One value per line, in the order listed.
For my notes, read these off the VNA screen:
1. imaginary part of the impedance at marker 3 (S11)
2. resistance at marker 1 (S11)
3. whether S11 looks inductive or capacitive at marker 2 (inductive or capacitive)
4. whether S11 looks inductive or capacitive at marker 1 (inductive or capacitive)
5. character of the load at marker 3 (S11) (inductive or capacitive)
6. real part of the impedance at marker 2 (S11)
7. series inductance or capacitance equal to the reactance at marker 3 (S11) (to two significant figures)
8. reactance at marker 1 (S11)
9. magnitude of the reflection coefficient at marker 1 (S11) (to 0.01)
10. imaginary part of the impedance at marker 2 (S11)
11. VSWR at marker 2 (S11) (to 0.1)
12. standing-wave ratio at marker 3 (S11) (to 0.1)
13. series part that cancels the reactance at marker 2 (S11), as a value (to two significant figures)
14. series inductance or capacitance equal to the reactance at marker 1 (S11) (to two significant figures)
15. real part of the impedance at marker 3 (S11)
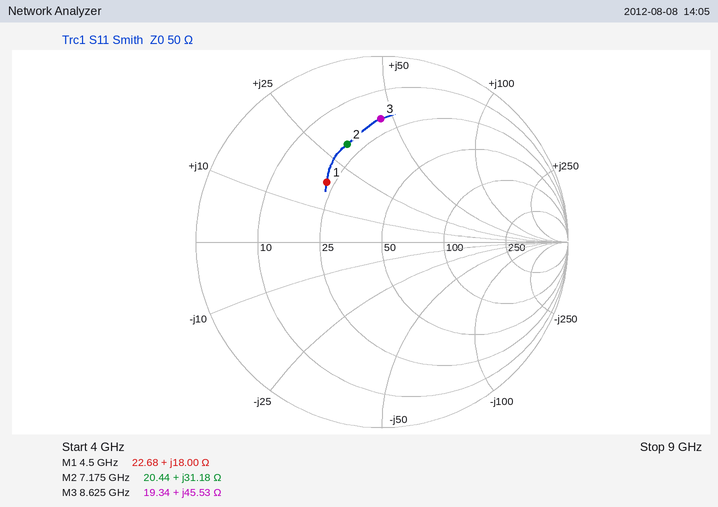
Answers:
+45.53 Ω
22.68 Ω
inductive
inductive
inductive
20.44 Ω
840 pH
+18.00 Ω
0.44
+31.18 Ω
3.5
4.9
710 fF
640 pH
19.34 Ω
